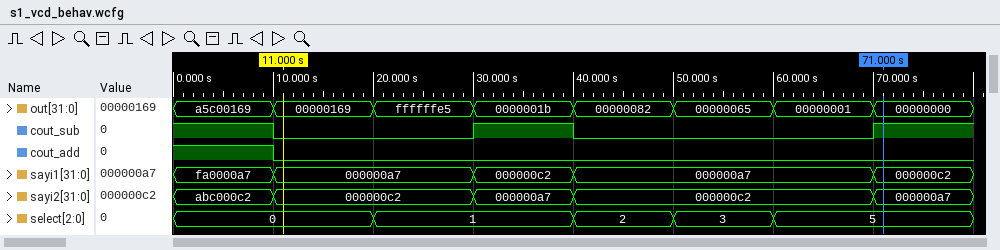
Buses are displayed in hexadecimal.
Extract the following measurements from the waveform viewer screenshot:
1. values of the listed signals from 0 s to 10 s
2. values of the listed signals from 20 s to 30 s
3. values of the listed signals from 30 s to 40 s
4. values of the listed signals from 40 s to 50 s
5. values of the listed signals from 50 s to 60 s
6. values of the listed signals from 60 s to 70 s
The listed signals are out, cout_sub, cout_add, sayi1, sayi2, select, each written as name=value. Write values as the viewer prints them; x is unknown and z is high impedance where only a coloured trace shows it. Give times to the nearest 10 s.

out=a5c00169, cout_sub=1, cout_add=1, sayi1=fa0000a7, sayi2=abc000c2, select=0
out=ffffffe5, cout_sub=0, cout_add=0, sayi1=000000a7, sayi2=000000c2, select=1
out=0000001b, cout_sub=1, cout_add=0, sayi1=000000c2, sayi2=000000a7, select=1
out=00000082, cout_sub=0, cout_add=0, sayi1=000000a7, sayi2=000000c2, select=2
out=00000065, cout_sub=0, cout_add=0, sayi1=000000a7, sayi2=000000c2, select=3
out=00000001, cout_sub=0, cout_add=0, sayi1=000000a7, sayi2=000000c2, select=5
